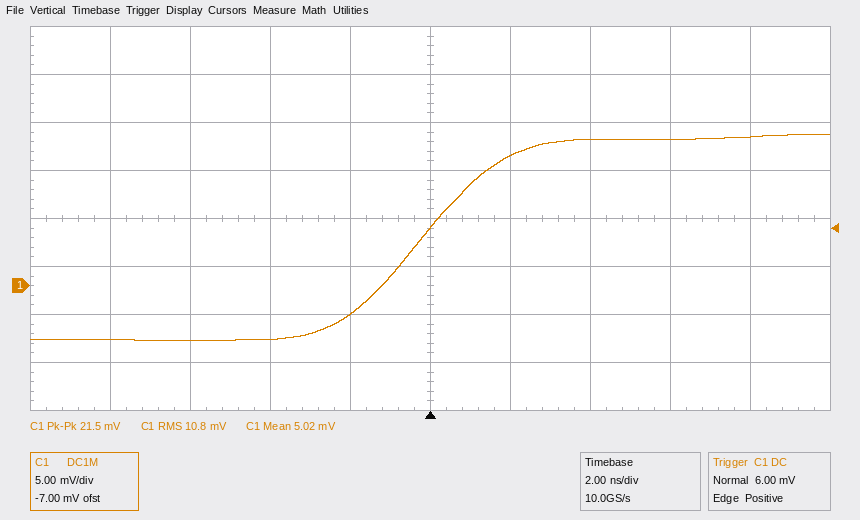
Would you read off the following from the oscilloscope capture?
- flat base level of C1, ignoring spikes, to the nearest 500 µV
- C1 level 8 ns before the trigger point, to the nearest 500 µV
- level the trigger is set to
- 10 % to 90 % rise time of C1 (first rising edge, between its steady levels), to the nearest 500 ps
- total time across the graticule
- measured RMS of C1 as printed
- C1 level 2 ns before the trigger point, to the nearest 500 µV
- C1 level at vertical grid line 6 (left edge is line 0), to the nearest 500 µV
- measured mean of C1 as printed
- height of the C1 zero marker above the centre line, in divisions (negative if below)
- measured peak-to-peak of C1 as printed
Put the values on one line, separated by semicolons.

-5.5 mV; -5.5 mV; 6.00 mV; 4.0 ns; 20 ns; 10.8 mV; -3.0 mV; 13.5 mV; 5.02 mV; -1.4 div; 21.5 mV
